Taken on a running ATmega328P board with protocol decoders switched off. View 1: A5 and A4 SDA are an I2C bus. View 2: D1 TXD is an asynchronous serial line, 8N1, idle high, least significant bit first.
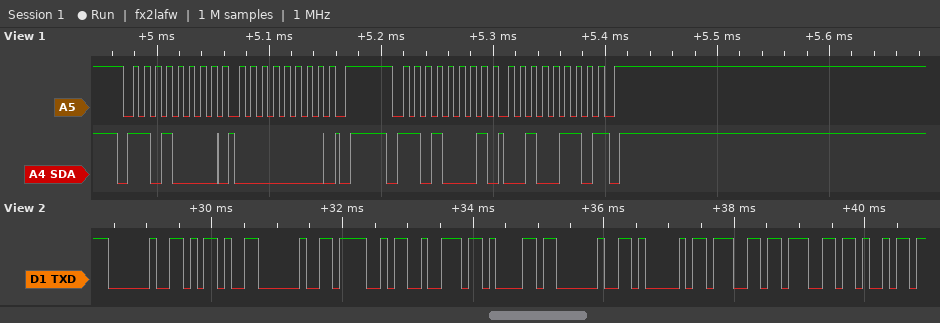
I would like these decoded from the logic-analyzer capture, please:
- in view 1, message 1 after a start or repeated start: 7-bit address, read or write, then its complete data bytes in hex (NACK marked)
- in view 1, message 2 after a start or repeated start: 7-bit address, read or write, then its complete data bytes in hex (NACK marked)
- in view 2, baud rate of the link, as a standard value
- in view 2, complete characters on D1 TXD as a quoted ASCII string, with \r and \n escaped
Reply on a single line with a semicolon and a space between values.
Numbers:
0x68 write: 00; 0x68 read: 26 NACK; 9600 baud; " - Ora Aggi"
